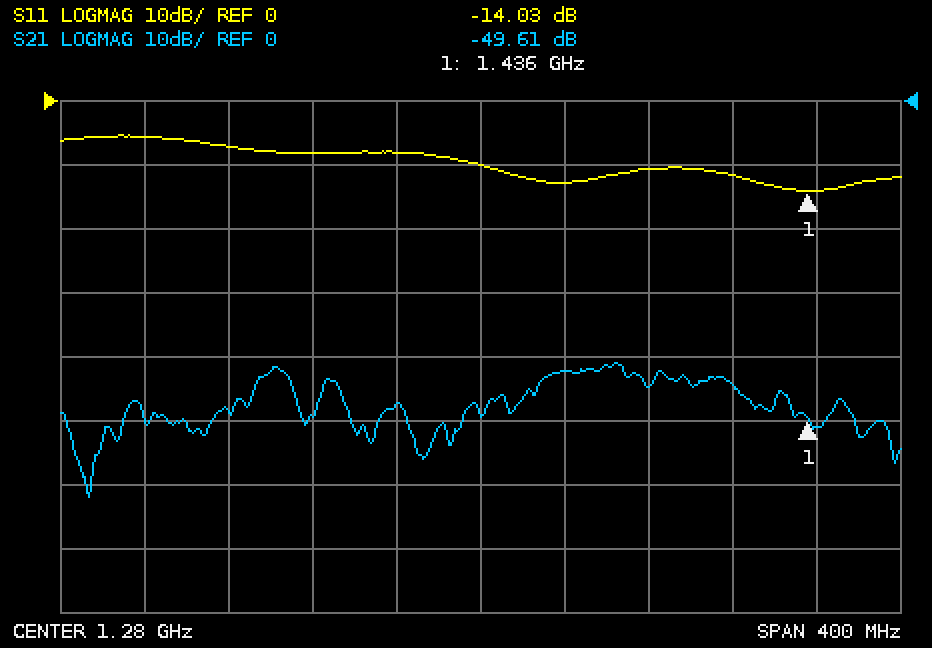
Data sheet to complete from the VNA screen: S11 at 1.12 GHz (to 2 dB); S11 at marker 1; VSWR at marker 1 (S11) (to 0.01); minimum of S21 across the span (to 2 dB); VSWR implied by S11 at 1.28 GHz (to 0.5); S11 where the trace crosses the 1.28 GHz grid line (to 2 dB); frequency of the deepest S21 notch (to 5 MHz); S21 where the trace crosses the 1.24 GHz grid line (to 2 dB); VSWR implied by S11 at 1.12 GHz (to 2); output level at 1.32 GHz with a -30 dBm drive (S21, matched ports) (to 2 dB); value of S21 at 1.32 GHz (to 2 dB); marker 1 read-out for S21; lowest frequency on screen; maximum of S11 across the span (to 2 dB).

-6 dB
-14.03 dB
1.50
-62 dB
2.0
-10 dB
1.095 GHz
-48 dB
4
-72 dBm
-42 dB
-49.61 dB
1.08 GHz
-6 dB
